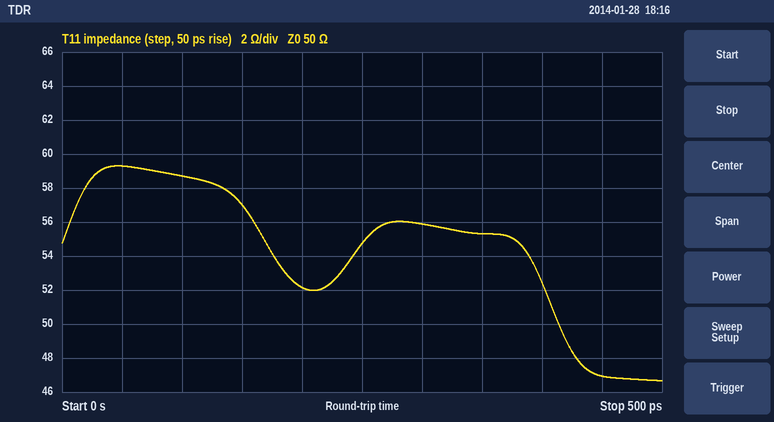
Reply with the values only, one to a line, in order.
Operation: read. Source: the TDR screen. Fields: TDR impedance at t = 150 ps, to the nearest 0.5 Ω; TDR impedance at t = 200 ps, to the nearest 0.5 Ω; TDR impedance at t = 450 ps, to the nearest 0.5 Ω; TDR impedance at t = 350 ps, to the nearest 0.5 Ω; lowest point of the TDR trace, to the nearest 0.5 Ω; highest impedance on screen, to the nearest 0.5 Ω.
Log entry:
57.0 Ω
52.0 Ω
47.0 Ω
55.5 Ω
46.5 Ω
59.5 Ω
